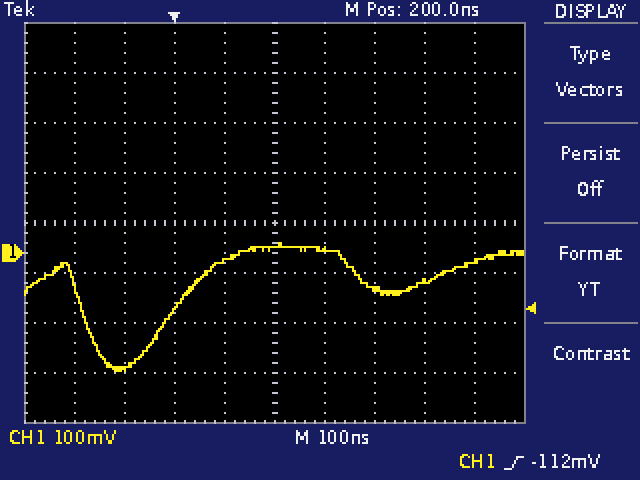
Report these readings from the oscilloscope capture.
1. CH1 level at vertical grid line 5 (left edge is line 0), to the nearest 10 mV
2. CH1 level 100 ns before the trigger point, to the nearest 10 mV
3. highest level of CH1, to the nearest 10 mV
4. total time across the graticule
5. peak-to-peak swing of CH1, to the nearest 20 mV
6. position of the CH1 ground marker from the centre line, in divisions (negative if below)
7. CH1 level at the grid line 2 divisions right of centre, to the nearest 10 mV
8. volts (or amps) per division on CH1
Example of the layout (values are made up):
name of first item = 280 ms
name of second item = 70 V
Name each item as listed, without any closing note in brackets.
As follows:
CH1 level at vertical grid line 5 (left edge is line 0), to the nearest 10 mV = 10 mV
CH1 level 100 ns before the trigger point, to the nearest 10 mV = -230 mV
highest level of CH1, to the nearest 10 mV = 20 mV
total time across the graticule = 1 µs
peak-to-peak swing of CH1, to the nearest 20 mV = 260 mV
position of the CH1 ground marker from the centre line, in divisions = -0.6 div
CH1 level at the grid line 2 divisions right of centre, to the nearest 10 mV = -70 mV
volts (or amps) per division on CH1 = 100 mV
